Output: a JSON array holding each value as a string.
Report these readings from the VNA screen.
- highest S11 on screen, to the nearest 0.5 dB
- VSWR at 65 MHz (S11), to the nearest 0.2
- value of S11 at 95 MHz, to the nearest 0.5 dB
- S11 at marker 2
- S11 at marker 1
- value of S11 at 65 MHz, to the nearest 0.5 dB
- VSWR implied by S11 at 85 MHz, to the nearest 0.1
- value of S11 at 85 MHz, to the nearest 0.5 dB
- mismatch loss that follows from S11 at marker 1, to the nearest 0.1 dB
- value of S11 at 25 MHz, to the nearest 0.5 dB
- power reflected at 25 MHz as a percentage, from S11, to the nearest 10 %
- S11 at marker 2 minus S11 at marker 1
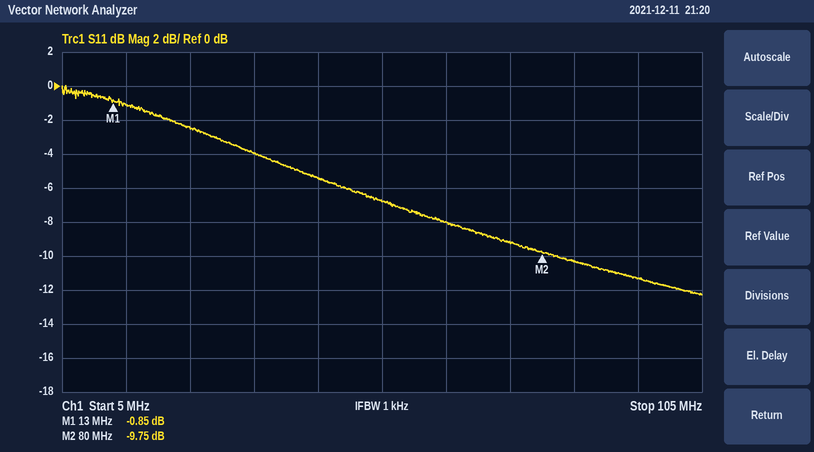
["0.0 dB", "2.4", "-11.5 dB", "-9.75 dB", "-0.85 dB", "-8.0 dB", "1.9", "-10.5 dB", "7.5 dB", "-2.5 dB", "60 %", "-8.90 dB"]
